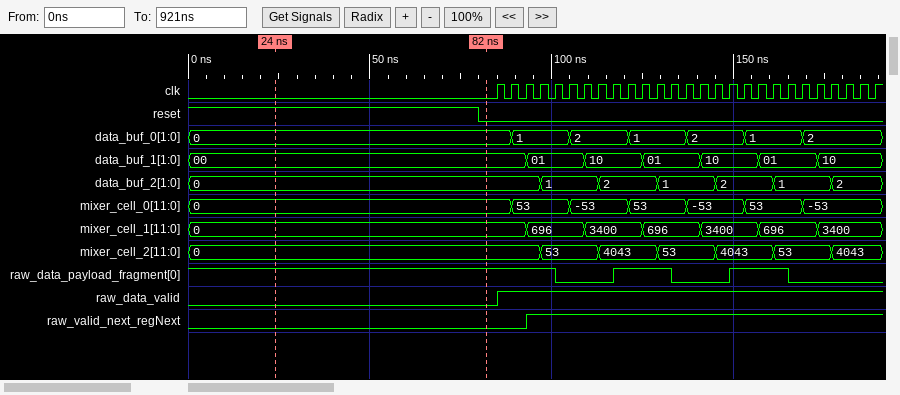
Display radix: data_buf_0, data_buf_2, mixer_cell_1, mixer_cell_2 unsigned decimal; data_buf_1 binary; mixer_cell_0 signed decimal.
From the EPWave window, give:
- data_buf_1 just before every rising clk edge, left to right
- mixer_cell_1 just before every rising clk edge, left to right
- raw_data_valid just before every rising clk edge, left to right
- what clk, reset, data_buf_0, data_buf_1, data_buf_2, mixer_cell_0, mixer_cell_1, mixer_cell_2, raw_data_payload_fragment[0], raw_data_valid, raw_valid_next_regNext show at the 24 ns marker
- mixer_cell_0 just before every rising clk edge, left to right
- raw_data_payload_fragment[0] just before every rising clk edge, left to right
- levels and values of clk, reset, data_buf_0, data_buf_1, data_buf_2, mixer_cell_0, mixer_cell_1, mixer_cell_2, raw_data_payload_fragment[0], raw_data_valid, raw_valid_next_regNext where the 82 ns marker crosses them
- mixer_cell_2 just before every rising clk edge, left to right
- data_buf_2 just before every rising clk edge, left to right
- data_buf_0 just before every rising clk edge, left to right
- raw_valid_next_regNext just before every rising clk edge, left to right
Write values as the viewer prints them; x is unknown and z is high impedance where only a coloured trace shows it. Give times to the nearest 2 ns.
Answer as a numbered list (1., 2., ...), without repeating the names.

1. 00, 00, 00, 01, 01, 01, 01, 10, 10, 10, 10, 01, 01, 01, 01, 10, 10, 10, 10, 01, 01, 01, 01, 10, 10, 10, 10
2. 0, 0, 0, 696, 696, 696, 696, 3400, 3400, 3400, 3400, 696, 696, 696, 696, 3400, 3400, 3400, 3400, 696, 696, 696, 696, 3400, 3400, 3400, 3400
3. 0 1 1 1 1 1 1 1 1 1 1 1 1 1 1 1 1 1 1 1 1 1 1 1 1 1 1
4. clk=0, reset=1, data_buf_0=0, data_buf_1=00, data_buf_2=0, mixer_cell_0=0, mixer_cell_1=0, mixer_cell_2=0, raw_data_payload_fragment[0]=1, raw_data_valid=0, raw_valid_next_regNext=0
5. 0, 0, 53, 53, 53, 53, -53, -53, -53, -53, 53, 53, 53, 53, -53, -53, -53, -53, 53, 53, 53, 53, -53, -53, -53, -53, -53
6. 1 1 1 1 1 0 0 0 0 1 1 1 1 0 0 0 0 1 1 1 1 0 0 0 0 0 0
7. clk=0, reset=0, data_buf_0=0, data_buf_1=00, data_buf_2=0, mixer_cell_0=0, mixer_cell_1=0, mixer_cell_2=0, raw_data_payload_fragment[0]=1, raw_data_valid=0, raw_valid_next_regNext=0
8. 0, 0, 0, 0, 53, 53, 53, 53, 4043, 4043, 4043, 4043, 53, 53, 53, 53, 4043, 4043, 4043, 4043, 53, 53, 53, 53, 4043, 4043, 4043
9. 0, 0, 0, 0, 1, 1, 1, 1, 2, 2, 2, 2, 1, 1, 1, 1, 2, 2, 2, 2, 1, 1, 1, 1, 2, 2, 2
10. 0, 0, 1, 1, 1, 1, 2, 2, 2, 2, 1, 1, 1, 1, 2, 2, 2, 2, 1, 1, 1, 1, 2, 2, 2, 2, 2
11. 0 0 0 1 1 1 1 1 1 1 1 1 1 1 1 1 1 1 1 1 1 1 1 1 1 1 1
